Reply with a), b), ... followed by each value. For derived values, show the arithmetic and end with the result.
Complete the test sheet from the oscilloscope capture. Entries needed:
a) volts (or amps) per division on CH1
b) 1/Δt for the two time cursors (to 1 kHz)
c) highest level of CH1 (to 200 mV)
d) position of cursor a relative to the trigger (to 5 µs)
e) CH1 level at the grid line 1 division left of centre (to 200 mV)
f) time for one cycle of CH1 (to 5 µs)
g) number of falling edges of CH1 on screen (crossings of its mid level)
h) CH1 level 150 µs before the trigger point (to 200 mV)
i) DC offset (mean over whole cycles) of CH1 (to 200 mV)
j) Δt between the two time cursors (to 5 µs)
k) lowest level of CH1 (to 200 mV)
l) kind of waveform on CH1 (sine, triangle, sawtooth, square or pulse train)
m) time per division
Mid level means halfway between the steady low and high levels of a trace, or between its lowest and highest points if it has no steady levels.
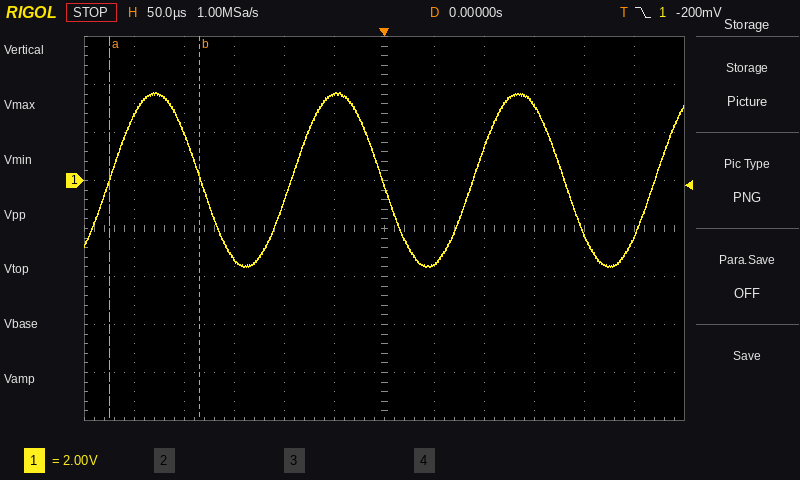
a) 2 V
b) 1 / 90 µs ≈ 11 kHz
c) 3.6 V
d) -275 µs
e) 3.6 V
f) 180 µs
g) 3
h) -3.2 V
i) (3.6 V + (-3.6 V)) / 2 ≈ 0.0 V
j) 90 µs
k) -3.6 V
l) sine
m) 50 µs
